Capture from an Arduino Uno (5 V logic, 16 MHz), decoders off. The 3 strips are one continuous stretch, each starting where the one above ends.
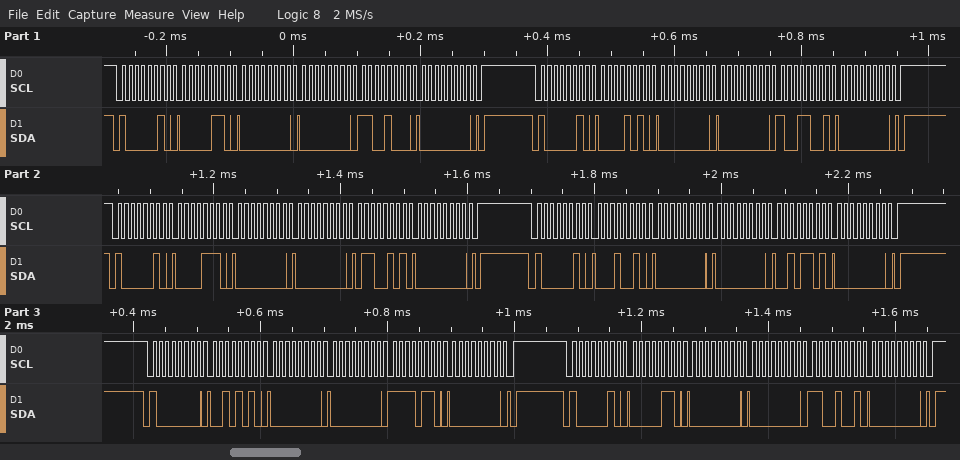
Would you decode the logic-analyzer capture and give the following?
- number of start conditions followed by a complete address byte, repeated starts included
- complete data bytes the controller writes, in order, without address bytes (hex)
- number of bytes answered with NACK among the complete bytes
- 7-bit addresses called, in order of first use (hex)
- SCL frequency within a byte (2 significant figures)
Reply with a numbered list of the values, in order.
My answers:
1. 6
2. 06 00 00 C8 00 0A 00 00 99 00 0E 00 00 65 00 12 00 00 2D 00 2A 00 00 F6 00 06 00 00 C9 00
3. 0
4. 0x41 0x40
5. 100 kHz
